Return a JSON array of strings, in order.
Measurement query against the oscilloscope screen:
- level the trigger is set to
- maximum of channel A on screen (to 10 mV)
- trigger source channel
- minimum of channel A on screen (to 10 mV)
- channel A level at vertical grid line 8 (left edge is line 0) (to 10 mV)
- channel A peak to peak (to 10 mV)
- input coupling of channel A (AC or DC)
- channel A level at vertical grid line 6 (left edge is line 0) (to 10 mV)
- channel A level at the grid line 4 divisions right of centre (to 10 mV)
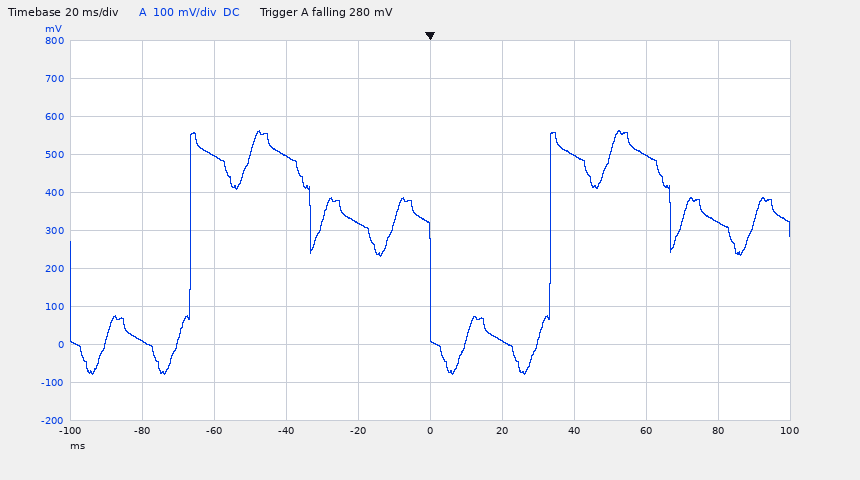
["280 mV", "560 mV", "channel A", "-80 mV", "500 mV", "640 mV", "DC", "10 mV", "320 mV"]
